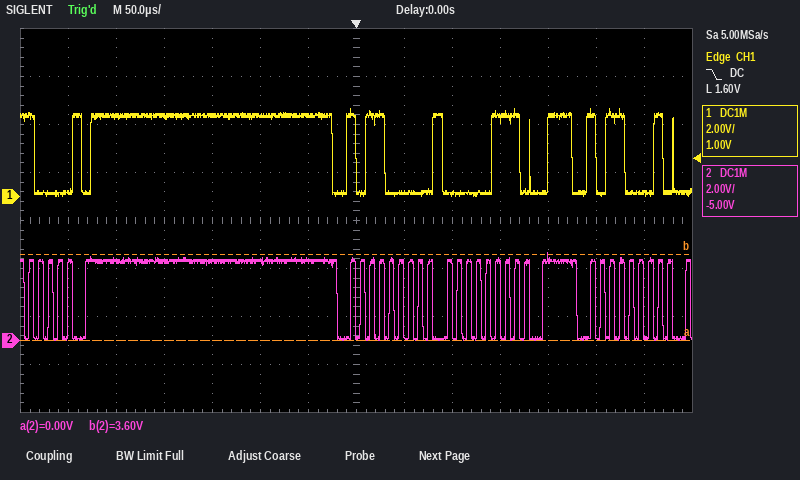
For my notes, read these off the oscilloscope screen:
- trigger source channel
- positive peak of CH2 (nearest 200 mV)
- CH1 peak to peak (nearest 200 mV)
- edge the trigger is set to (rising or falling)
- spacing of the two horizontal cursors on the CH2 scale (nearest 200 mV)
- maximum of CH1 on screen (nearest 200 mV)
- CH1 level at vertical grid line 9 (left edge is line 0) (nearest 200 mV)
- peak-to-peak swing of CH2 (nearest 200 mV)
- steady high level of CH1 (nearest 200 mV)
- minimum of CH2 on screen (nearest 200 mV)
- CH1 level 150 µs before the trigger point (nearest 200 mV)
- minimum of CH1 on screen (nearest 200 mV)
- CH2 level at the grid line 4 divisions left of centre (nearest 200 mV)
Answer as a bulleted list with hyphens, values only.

- CH1
- 3.6 V
- 3.6 V
- falling
- 3.6 V
- 3.6 V
- 200 mV
- 3.6 V
- 3.4 V
- 0.0 V
- 3.4 V
- 0.0 V
- 3.2 V
